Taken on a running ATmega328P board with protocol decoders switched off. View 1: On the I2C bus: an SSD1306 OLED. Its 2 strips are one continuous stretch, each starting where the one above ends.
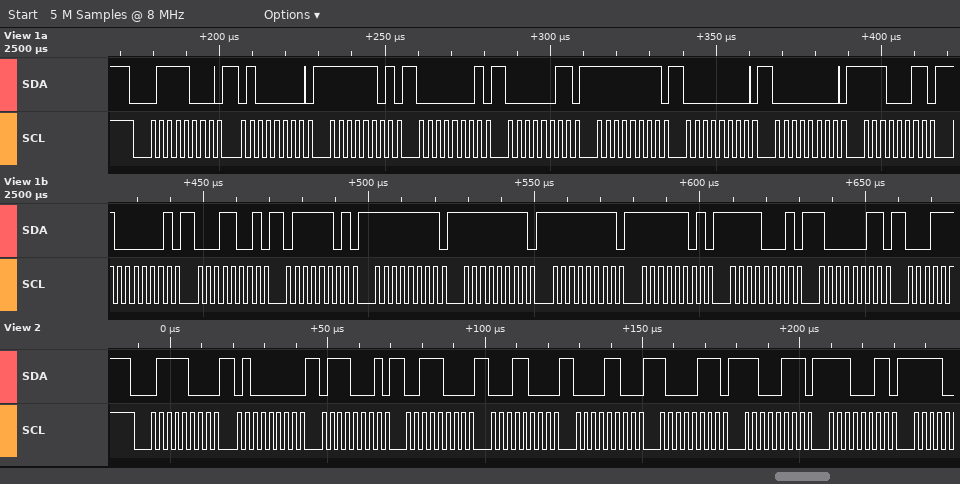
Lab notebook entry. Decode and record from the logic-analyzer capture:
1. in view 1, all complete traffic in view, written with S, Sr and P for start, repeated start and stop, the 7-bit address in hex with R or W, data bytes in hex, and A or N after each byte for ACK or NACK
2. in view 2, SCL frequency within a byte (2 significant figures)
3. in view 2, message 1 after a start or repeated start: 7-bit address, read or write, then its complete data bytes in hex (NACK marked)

S 3CW A 40 A FD A 01 A 03 A FF A 00 A 00 A E3 A 81 A 19 A 7D A FF A FF A FF A FD A F1 A 83 A
400 kHz
0x3C write: 40 71 38 18 0C 87 C7 E3
